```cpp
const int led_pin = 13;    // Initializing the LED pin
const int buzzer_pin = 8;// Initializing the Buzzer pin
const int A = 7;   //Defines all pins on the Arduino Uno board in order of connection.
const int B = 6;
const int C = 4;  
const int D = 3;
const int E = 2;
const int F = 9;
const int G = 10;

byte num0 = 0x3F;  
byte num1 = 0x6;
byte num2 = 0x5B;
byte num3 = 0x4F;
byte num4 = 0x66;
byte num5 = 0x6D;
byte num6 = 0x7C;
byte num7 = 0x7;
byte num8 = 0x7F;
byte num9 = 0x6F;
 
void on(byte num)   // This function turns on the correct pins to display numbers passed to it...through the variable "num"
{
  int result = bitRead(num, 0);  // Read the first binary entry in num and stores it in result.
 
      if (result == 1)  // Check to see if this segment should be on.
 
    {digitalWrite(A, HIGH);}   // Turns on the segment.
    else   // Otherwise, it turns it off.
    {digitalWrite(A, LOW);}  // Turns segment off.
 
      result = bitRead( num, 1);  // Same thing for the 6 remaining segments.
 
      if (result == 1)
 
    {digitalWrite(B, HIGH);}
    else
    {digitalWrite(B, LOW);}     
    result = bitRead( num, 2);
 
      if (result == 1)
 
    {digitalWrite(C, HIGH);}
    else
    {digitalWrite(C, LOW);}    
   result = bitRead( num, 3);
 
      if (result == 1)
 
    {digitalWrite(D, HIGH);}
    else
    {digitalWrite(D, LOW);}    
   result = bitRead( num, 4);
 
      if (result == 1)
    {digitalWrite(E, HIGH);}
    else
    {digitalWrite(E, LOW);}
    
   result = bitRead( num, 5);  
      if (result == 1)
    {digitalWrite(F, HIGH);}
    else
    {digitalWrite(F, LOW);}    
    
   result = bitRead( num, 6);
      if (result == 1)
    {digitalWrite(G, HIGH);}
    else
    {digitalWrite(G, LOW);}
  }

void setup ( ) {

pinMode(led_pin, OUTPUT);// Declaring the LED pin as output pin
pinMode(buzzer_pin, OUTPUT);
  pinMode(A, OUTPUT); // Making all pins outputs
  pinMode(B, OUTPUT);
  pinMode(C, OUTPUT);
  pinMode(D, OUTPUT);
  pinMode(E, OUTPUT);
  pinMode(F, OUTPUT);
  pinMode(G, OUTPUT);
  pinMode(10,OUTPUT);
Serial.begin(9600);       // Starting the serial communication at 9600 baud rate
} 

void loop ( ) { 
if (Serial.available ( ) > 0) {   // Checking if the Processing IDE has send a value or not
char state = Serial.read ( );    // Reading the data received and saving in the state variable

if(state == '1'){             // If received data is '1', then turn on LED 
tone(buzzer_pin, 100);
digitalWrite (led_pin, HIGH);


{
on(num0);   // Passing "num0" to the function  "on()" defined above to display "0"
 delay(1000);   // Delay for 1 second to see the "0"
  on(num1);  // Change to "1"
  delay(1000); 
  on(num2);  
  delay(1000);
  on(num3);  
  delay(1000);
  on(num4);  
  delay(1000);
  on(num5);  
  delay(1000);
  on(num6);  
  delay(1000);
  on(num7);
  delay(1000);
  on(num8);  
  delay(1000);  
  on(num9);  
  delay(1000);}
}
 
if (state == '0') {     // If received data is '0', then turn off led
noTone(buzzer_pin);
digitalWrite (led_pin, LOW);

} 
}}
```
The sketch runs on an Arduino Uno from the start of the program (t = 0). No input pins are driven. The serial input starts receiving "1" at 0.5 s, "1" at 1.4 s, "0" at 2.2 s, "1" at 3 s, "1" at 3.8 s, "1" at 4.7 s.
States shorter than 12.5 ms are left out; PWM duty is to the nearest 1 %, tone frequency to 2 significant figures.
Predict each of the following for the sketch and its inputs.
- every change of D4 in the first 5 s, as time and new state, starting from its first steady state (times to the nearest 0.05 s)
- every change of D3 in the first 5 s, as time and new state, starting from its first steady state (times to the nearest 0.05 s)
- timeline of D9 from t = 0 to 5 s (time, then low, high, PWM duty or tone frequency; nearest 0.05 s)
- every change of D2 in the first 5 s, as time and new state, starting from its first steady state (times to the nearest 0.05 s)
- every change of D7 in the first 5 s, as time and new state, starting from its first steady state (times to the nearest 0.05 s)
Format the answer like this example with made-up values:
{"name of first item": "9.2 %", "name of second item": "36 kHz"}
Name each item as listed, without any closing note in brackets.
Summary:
{"every change of D4 in the first 5 s, as time and new state, starting from its first steady state": "0 s low; 0.5 s high; 2.5 s low; 3.5 s high", "every change of D3 in the first 5 s, as time and new state, starting from its first steady state": "0 s low; 0.5 s high; 1.5 s low; 2.5 s high; 4.5 s low", "timeline of D9 from t = 0 to 5 s": "0 s low; 0.5 s high; 1.5 s low; 4.5 s high", "every change of D2 in the first 5 s, as time and new state, starting from its first steady state": "0 s low; 0.5 s high; 1.5 s low; 2.5 s high; 3.5 s low", "every change of D7 in the first 5 s, as time and new state, starting from its first steady state": "0 s low; 0.5 s high; 1.5 s low; 2.5 s high; 4.5 s low"}
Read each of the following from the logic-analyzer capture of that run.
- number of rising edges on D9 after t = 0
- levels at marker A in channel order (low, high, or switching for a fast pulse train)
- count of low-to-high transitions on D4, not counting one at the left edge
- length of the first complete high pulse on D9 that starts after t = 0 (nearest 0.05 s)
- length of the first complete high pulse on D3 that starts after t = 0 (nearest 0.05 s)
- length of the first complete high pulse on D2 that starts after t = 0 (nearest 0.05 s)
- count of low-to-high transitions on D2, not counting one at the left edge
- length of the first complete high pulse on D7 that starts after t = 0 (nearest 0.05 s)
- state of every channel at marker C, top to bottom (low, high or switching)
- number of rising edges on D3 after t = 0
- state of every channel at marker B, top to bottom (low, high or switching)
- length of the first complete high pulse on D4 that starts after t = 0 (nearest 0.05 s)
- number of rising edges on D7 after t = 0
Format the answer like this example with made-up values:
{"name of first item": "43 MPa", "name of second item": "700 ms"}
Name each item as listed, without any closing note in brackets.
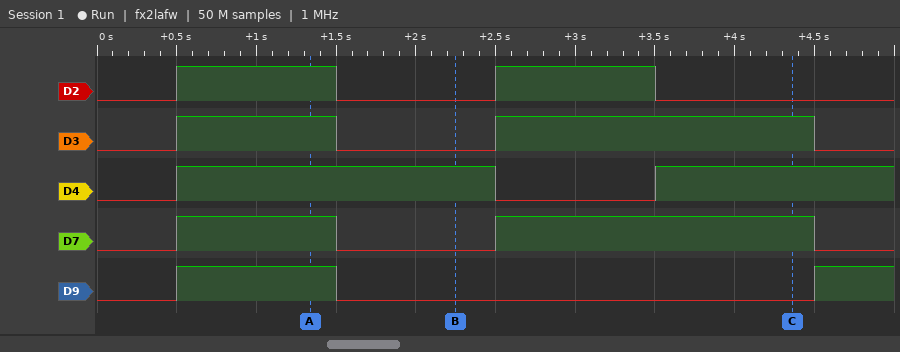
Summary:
{"number of rising edges on D9 after t = 0": "2", "levels at marker A in channel order": "D2 high, D3 high, D4 high, D7 high, D9 high", "count of low-to-high transitions on D4, not counting one at the left edge": "2", "length of the first complete high pulse on D9 that starts after t = 0": "1.00 s", "length of the first complete high pulse on D3 that starts after t = 0": "1.00 s", "length of the first complete high pulse on D2 that starts after t = 0": "1.00 s", "count of low-to-high transitions on D2, not counting one at the left edge": "2", "length of the first complete high pulse on D7 that starts after t = 0": "1.00 s", "state of every channel at marker C, top to bottom": "D2 low, D3 high, D4 high, D7 high, D9 low", "number of rising edges on D3 after t = 0": "2", "state of every channel at marker B, top to bottom": "D2 low, D3 low, D4 high, D7 low, D9 low", "length of the first complete high pulse on D4 that starts after t = 0": "2.00 s", "number of rising edges on D7 after t = 0": "2"}
